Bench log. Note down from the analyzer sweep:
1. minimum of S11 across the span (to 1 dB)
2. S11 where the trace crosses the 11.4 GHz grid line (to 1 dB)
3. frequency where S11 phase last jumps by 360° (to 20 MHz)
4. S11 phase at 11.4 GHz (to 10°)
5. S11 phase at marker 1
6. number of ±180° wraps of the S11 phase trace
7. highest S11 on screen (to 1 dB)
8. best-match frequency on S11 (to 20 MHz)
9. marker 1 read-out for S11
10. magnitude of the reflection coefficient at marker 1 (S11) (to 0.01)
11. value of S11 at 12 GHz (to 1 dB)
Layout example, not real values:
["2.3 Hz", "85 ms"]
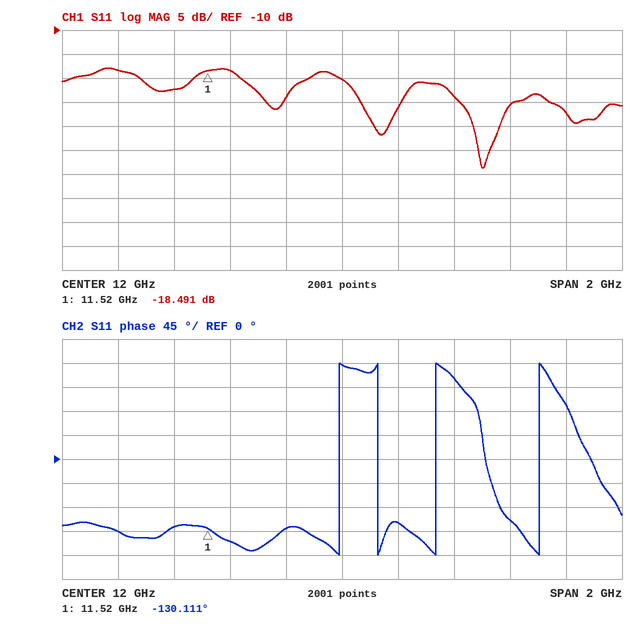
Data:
["-39 dB", "-22 dB", "12.70 GHz", "-130°", "-130.111°", "4", "-18 dB", "12.50 GHz", "-18.491 dB", "0.12", "-20 dB"]
